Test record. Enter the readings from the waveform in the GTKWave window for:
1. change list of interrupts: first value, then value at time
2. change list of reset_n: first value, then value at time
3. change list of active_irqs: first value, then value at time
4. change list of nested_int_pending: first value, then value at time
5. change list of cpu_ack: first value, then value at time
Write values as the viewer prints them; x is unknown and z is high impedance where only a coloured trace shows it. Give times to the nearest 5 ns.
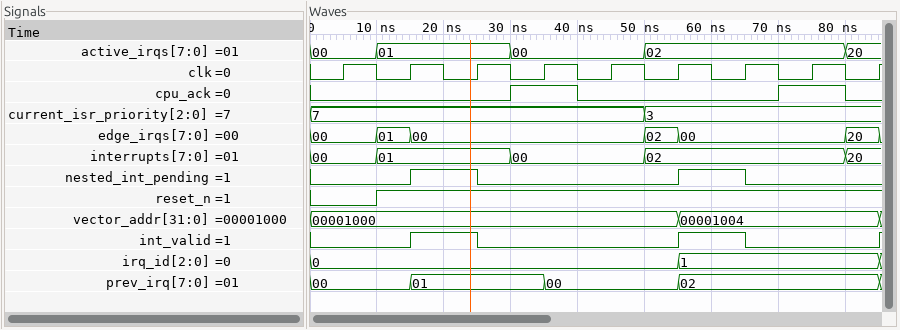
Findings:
00, 01 at 10 ns, 00 at 30 ns, 02 at 50 ns, 20 at 80 ns
0, 1 at 10 ns
00, 01 at 10 ns, 00 at 30 ns, 02 at 50 ns, 20 at 80 ns
0, 1 at 15 ns, 0 at 25 ns, 1 at 55 ns, 0 at 65 ns
0, 1 at 30 ns, 0 at 40 ns, 1 at 70 ns, 0 at 80 ns
